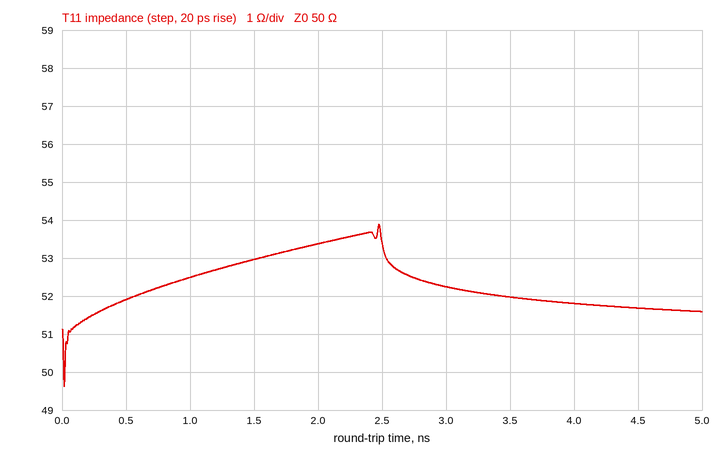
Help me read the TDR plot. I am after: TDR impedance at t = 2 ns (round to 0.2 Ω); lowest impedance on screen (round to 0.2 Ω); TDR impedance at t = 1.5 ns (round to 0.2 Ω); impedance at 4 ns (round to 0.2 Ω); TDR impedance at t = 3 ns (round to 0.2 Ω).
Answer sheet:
53.4 Ω
49.6 Ω
53.0 Ω
51.8 Ω
52.2 Ω
